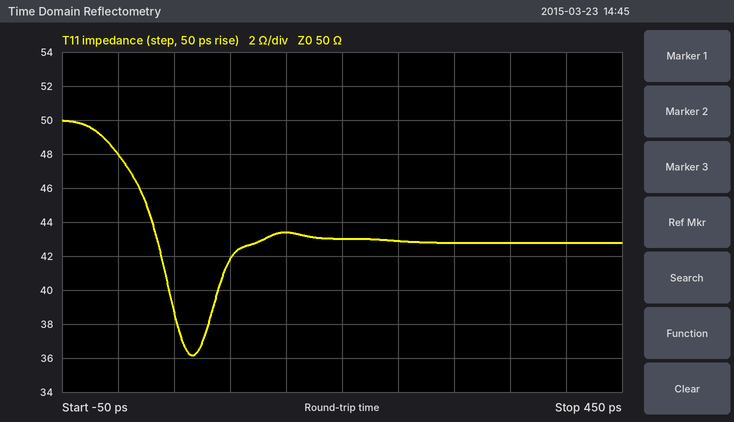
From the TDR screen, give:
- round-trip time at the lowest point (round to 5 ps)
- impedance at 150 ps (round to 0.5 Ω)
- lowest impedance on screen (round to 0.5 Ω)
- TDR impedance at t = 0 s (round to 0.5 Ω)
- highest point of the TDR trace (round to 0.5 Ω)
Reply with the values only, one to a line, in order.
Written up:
65 ps
43.5 Ω
36.0 Ω
48.0 Ω
50.0 Ω
